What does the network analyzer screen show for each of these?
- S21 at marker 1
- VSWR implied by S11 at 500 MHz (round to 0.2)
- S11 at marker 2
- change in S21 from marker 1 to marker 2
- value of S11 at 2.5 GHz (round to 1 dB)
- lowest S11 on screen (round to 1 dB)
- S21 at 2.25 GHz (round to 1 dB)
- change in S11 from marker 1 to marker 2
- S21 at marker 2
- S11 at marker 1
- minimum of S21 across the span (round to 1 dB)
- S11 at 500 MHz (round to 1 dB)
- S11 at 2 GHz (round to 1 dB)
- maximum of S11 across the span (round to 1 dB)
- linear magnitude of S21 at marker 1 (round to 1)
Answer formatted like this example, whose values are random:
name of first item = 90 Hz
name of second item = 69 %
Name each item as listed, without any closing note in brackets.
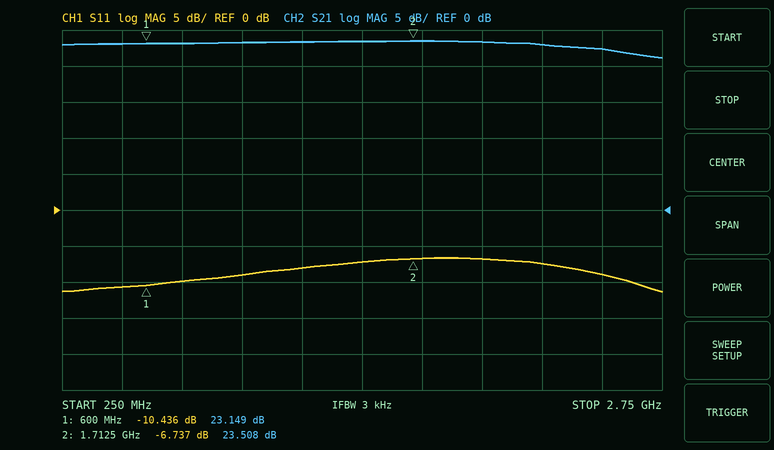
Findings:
S21 at marker 1 = 23.149 dB
VSWR implied by S11 at 500 MHz = 1.8
S11 at marker 2 = -6.737 dB
change in S21 from marker 1 to marker 2 = 0.359 dB
value of S11 at 2.5 GHz = -9 dB
lowest S11 on screen = -11 dB
S21 at 2.25 GHz = 23 dB
change in S11 from marker 1 to marker 2 = 3.699 dB
S21 at marker 2 = 23.508 dB
S11 at marker 1 = -10.436 dB
minimum of S21 across the span = 21 dB
S11 at 500 MHz = -11 dB
S11 at 2 GHz = -7 dB
maximum of S11 across the span = -7 dB
linear magnitude of S21 at marker 1 = 14
